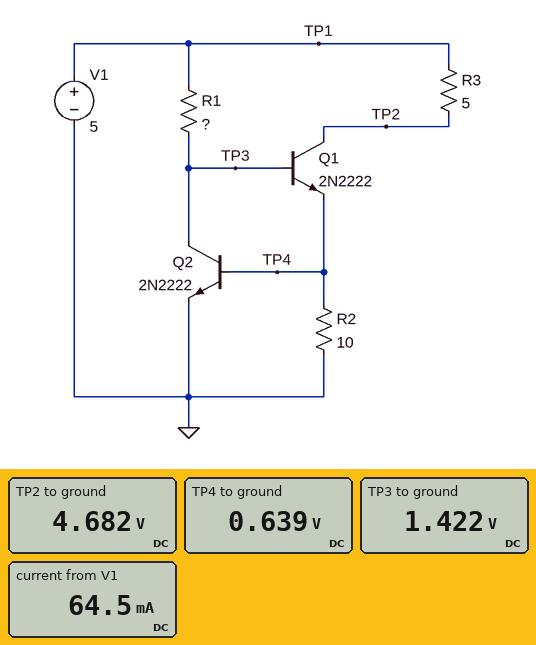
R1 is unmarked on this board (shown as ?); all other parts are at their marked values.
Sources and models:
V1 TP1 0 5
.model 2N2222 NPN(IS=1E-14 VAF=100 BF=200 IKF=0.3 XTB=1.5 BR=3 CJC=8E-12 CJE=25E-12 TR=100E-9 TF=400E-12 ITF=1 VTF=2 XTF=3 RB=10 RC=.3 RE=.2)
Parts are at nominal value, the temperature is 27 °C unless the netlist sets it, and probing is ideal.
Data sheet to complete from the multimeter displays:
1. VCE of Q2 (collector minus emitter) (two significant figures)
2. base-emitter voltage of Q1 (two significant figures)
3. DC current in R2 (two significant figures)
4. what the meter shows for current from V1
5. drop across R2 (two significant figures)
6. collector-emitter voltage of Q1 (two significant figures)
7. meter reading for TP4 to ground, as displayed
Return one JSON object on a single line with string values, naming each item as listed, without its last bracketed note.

{"VCE of Q2 (collector minus emitter)": "1.4 V", "base-emitter voltage of Q1": "780 mV", "DC current in R2": "64 mA", "what the meter shows for current from V1": "64.5 mA", "drop across R2": "640 mV", "collector-emitter voltage of Q1": "4.0 V", "meter reading for TP4 to ground, as displayed": "0.639 V"}
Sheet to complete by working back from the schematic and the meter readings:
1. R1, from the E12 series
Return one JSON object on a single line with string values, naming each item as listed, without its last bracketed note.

{"R1, from the E12 series": "3.9 kΩ"}
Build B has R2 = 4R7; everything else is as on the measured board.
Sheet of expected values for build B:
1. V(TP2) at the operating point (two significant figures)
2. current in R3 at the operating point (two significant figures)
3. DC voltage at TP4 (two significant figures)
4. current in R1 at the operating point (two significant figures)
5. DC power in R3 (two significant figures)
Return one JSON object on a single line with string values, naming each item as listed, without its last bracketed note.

{"V(TP2) at the operating point": "4.4 V", "current in R3 at the operating point": "120 mA", "DC voltage at TP4": "590 mV", "current in R1 at the operating point": "920 µA", "DC power in R3": "77 mW"}
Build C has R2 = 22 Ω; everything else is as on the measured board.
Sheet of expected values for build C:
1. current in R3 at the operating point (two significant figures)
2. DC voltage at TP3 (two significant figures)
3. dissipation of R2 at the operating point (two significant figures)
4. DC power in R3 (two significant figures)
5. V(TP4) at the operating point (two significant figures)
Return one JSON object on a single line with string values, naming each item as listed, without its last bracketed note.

{"current in R3 at the operating point": "29 mA", "DC voltage at TP3": "1.4 V", "dissipation of R2 at the operating point": "19 mW", "DC power in R3": "4.3 mW", "V(TP4) at the operating point": "650 mV"}
